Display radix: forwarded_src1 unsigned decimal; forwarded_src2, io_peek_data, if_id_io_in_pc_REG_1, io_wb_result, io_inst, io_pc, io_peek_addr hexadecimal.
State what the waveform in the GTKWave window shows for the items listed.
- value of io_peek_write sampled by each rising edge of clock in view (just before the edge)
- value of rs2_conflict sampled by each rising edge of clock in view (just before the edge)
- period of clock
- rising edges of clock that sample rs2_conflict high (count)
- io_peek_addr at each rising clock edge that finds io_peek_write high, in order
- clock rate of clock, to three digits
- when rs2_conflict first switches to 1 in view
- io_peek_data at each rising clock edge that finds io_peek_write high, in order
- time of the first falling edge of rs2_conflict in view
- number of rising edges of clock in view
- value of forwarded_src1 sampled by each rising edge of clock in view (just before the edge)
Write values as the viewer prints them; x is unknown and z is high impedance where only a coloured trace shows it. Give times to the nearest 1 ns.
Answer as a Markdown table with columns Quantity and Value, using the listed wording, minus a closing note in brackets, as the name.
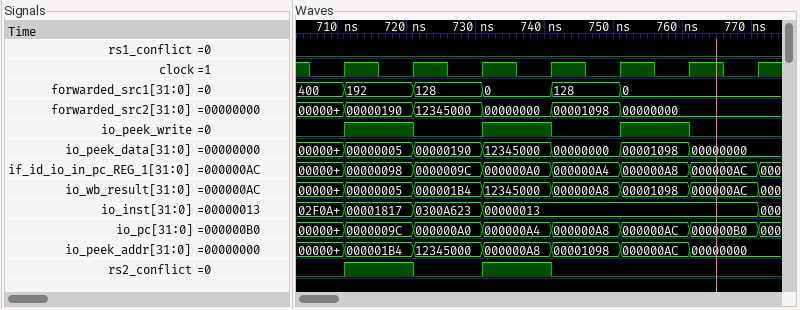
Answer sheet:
| Quantity | Value |
|---|---|
| value of io_peek_write sampled by each rising edge of clock in view | 0 1 0 1 0 1 0 |
| value of rs2_conflict sampled by each rising edge of clock in view | 0 1 0 1 0 0 0 |
| period of clock | 10 ns |
| rising edges of clock that sample rs2_conflict high | 2 |
| io_peek_addr at each rising clock edge that finds io_peek_write high, in order | 000001B4, 000000A8, 000000AC |
| clock rate of clock, to three digits | 100 MHz |
| when rs2_conflict first switches to 1 in view | 711 ns |
| io_peek_data at each rising clock edge that finds io_peek_write high, in order | 00000005, 12345000, 00001098 |
| time of the first falling edge of rs2_conflict in view | 721 ns |
| number of rising edges of clock in view | 7 |
| value of forwarded_src1 sampled by each rising edge of clock in view | 400, 192, 128, 0, 128, 0, 0 |
